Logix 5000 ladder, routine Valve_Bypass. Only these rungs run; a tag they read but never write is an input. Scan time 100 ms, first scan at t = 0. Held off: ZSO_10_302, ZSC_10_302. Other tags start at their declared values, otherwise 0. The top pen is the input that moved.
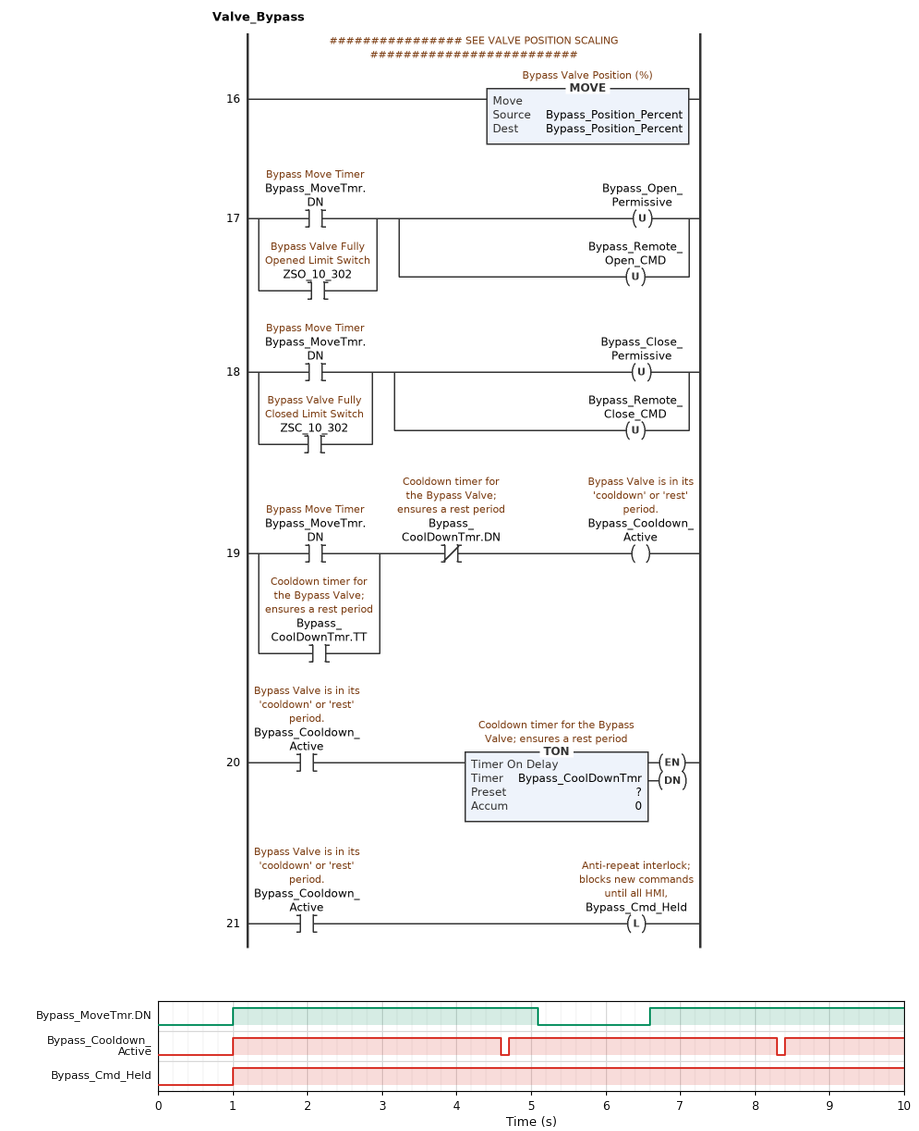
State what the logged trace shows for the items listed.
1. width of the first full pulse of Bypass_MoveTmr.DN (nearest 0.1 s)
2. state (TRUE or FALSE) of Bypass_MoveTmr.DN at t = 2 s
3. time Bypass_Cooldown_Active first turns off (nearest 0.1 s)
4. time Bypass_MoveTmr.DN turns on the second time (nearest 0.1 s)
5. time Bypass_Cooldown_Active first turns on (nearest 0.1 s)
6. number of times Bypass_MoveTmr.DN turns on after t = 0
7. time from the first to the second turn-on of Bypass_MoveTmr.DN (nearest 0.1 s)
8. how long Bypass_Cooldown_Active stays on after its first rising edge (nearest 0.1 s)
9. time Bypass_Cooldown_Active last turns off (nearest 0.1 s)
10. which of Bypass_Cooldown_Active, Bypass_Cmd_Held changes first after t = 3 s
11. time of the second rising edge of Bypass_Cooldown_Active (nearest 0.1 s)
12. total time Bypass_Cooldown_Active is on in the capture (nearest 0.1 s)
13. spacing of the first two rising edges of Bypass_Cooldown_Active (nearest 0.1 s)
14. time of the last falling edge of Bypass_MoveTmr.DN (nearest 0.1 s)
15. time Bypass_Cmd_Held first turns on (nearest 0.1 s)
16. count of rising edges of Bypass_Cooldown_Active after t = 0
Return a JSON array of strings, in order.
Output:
["4.1 s", "TRUE", "4.6 s", "6.6 s", "1.0 s", "2", "5.6 s", "3.6 s", "8.3 s", "Bypass_Cooldown_Active", "4.7 s", "8.8 s", "3.7 s", "5.1 s", "1.0 s", "3"]
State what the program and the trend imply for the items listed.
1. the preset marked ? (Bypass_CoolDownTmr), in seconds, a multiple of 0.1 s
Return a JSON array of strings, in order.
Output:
["3.5 s"]
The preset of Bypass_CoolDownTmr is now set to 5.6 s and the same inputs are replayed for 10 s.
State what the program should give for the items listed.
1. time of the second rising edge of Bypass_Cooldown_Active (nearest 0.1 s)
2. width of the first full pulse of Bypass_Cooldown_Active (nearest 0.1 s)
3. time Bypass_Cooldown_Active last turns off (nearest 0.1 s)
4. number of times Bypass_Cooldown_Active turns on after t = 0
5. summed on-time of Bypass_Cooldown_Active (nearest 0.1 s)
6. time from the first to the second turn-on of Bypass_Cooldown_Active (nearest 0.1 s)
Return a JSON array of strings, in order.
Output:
["6.8 s", "5.7 s", "6.7 s", "2", "8.9 s", "5.8 s"]
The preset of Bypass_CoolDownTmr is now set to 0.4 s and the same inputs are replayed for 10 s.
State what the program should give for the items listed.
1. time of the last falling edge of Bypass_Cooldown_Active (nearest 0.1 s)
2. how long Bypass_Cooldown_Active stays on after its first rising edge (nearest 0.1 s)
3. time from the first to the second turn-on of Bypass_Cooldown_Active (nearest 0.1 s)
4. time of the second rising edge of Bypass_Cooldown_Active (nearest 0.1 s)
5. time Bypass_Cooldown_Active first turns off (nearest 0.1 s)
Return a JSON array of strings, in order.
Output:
["9.5 s", "0.5 s", "0.6 s", "1.6 s", "1.5 s"]
